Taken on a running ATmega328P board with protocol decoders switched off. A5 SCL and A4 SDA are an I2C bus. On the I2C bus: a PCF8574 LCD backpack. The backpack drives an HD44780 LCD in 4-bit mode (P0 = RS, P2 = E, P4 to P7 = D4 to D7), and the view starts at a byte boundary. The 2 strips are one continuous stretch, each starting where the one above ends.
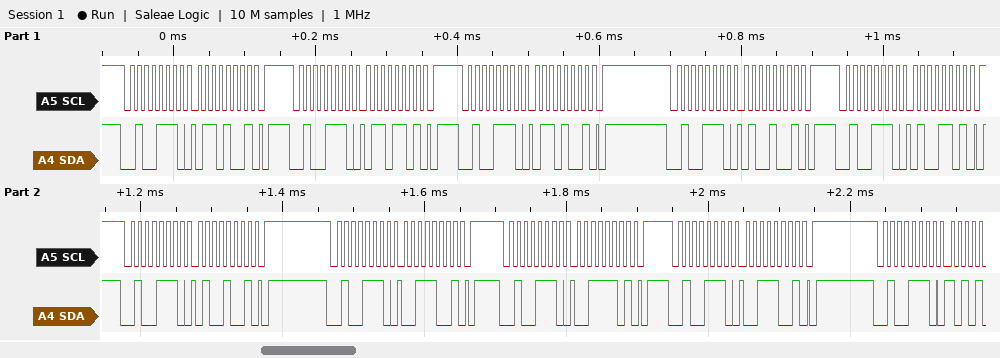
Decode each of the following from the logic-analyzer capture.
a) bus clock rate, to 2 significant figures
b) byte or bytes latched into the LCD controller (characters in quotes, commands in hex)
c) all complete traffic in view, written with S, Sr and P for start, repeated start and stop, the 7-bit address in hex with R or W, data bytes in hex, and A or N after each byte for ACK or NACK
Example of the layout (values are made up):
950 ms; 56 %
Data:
100 kHz; 'd'; S 27W A 69 A P S 27W A 6D A P S 27W A 69 A P S 27W A 49 A P S 27W A 4D A P S 27W A 49 A P S 27W A 39 A P S 27W A 3D A P S 27W A 39 A P S 27W A
